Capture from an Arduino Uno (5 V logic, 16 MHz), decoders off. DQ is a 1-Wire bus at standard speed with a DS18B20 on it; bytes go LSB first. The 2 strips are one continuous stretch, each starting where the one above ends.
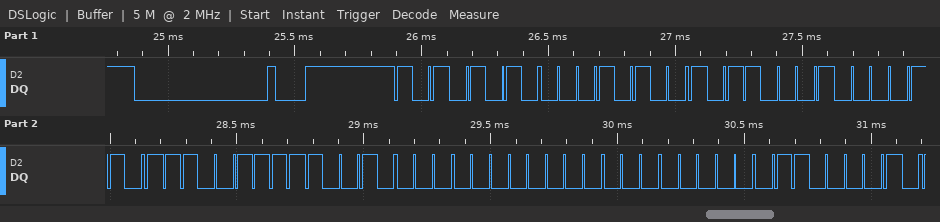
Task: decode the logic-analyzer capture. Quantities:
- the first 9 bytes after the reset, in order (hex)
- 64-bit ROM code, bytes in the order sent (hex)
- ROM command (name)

55 28 8D B0 F3 09 00 00 86
28 8D B0 F3 09 00 00 86
Match ROM
